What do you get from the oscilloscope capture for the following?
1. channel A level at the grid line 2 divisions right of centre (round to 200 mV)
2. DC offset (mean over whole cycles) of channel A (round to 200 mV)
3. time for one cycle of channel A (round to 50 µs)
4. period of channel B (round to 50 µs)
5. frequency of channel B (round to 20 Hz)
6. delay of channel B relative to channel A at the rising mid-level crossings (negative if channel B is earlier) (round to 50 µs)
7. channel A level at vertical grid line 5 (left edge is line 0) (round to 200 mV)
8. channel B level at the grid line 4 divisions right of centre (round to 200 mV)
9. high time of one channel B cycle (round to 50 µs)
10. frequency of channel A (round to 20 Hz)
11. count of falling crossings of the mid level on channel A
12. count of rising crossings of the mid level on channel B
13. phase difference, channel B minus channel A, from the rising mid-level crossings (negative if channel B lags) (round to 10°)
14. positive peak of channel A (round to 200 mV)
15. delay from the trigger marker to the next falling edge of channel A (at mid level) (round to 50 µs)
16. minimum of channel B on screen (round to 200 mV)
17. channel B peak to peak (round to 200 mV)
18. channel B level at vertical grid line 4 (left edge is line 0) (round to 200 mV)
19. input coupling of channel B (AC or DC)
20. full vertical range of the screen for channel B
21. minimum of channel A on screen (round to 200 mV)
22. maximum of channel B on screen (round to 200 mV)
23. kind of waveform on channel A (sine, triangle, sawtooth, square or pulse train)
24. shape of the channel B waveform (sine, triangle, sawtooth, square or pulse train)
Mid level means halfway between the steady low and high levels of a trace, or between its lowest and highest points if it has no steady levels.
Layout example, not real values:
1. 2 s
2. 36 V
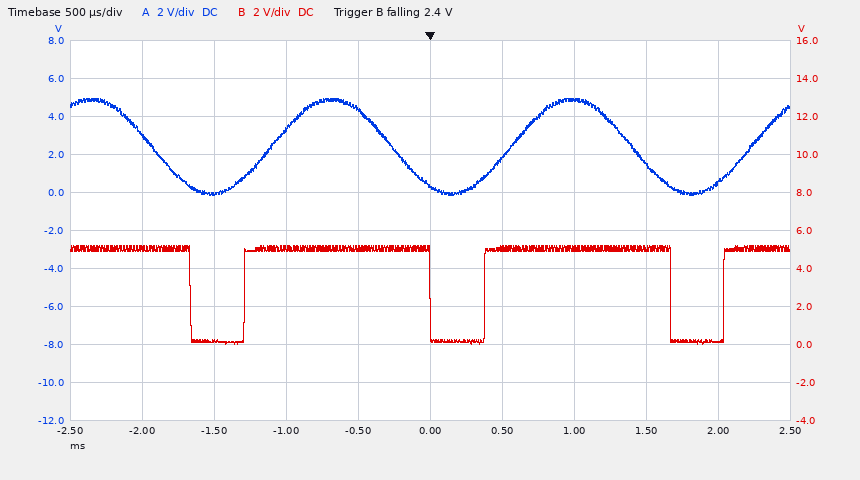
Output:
1. 4.8 V
2. 2.4 V
3. 1.65 ms
4. 1.65 ms
5. 600 Hz
6. -200 µs
7. 400 mV
8. 200 mV
9. 1.30 ms
10. 600 Hz
11. 3
12. 3
13. +40°
14. 5.0 V
15. 1.40 ms
16. 0.0 V
17. 5.2 V
18. 5.0 V
19. DC
20. 20 V
21. -200 mV
22. 5.2 V
23. sine
24. pulse train
